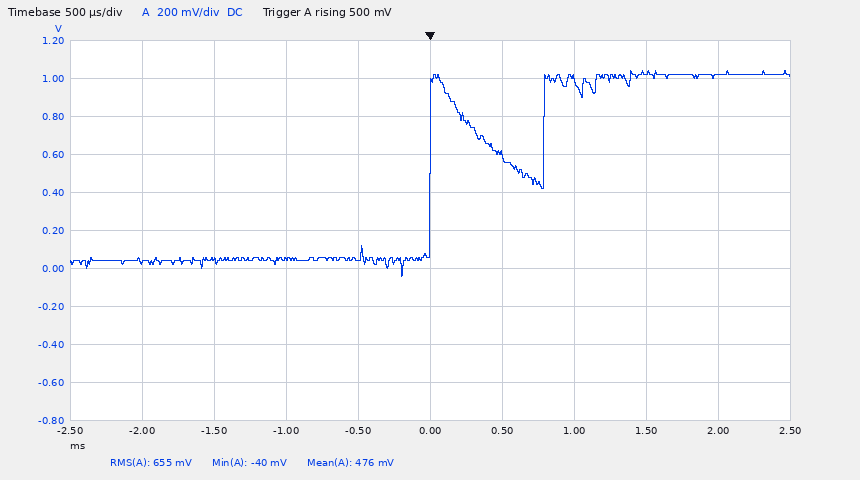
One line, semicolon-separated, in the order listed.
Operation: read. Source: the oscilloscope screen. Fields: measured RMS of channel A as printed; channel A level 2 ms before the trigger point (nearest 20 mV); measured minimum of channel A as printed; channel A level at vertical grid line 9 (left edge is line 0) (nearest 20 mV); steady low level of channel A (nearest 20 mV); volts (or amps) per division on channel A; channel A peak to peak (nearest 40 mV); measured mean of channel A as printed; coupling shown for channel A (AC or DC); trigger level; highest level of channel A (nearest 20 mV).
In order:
655 mV; 40 mV; -40 mV; 1.02 V; 40 mV; 200 mV; 1.08 V; 476 mV; DC; 500 mV; 1.04 V
